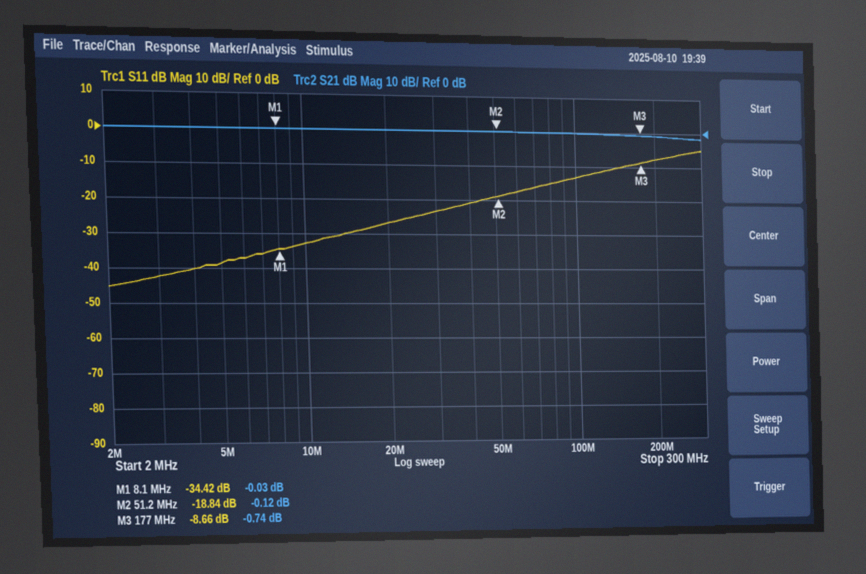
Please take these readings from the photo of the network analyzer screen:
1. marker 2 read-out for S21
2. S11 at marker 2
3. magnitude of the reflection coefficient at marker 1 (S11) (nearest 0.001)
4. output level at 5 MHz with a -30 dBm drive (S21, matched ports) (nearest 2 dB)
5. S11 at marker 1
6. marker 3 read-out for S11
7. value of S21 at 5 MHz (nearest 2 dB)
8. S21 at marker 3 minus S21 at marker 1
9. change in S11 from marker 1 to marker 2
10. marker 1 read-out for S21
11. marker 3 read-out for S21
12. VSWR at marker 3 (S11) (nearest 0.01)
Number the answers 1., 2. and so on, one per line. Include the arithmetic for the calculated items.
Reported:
1. -0.12 dB
2. -18.84 dB
3. 10^(-34.42/20) ≈ 0.019
4. -30 dBm + (0 dB) = -30 dBm
5. -34.42 dB
6. -8.66 dB
7. 0 dB
8. -0.74 − (-0.03) = -0.71 dB
9. -18.84 − (-34.42) = 15.58 dB
10. -0.03 dB
11. -0.74 dB
12. (1 + 0.3690)/(1 − 0.3690) ≈ 2.17
